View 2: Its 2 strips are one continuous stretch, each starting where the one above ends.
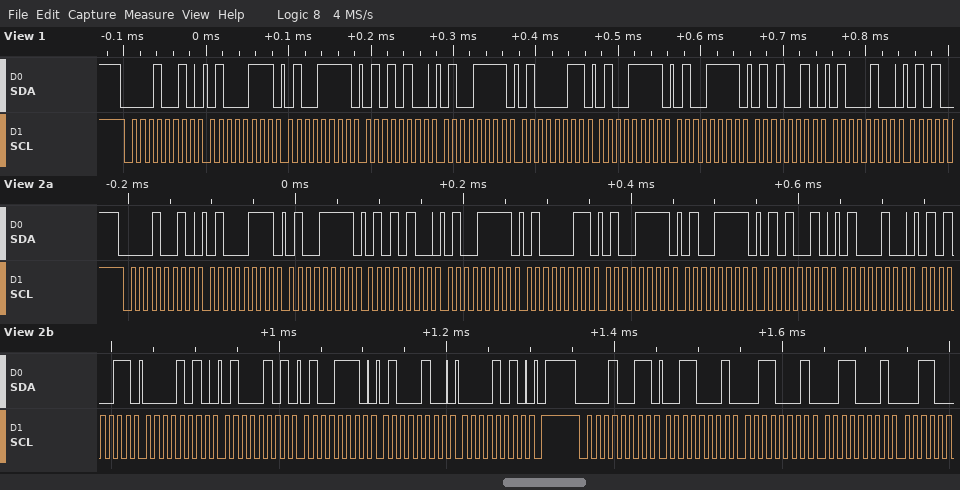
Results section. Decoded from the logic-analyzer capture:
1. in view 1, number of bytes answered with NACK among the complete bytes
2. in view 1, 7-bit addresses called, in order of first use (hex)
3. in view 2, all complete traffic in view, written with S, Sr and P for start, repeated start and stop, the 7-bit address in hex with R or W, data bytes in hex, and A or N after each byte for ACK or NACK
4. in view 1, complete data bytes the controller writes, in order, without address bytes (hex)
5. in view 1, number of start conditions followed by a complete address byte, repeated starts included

0
0x09
S 09W A 47 A 4F A 54 A 4F A 43 A 4F A 4F A 52 A 44 A 53 A 0A A 45 A 4E A 44 A 0A A P S 09R A 31 A 31 A 31 A
47 4F 54 4F 43 4F 4F 52 44
1
